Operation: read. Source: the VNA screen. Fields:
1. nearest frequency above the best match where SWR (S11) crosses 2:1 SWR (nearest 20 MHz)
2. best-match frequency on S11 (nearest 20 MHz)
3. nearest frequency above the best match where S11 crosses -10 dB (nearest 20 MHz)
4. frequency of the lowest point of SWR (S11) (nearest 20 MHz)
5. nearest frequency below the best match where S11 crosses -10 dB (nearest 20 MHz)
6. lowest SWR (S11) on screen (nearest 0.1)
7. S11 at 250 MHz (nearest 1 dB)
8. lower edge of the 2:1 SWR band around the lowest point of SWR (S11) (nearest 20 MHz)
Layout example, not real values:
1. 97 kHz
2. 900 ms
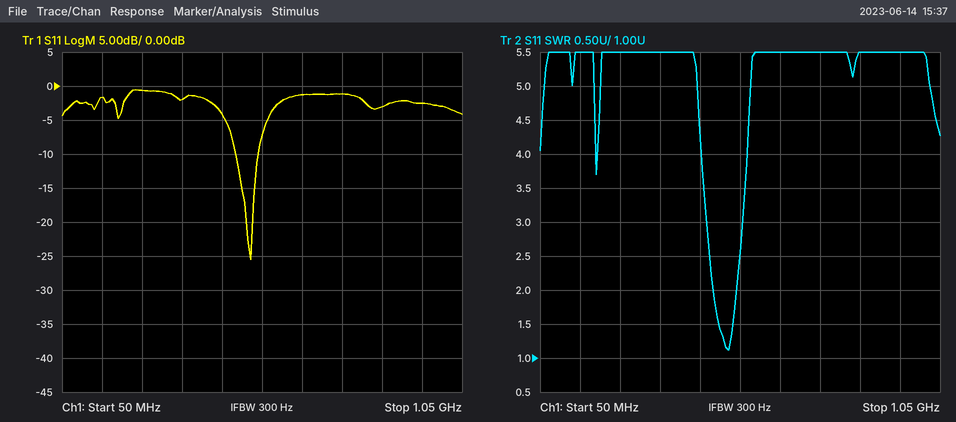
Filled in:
1. 540 MHz
2. 520 MHz
3. 540 MHz
4. 520 MHz
5. 480 MHz
6. 1.1
7. -1 dB
8. 480 MHz
